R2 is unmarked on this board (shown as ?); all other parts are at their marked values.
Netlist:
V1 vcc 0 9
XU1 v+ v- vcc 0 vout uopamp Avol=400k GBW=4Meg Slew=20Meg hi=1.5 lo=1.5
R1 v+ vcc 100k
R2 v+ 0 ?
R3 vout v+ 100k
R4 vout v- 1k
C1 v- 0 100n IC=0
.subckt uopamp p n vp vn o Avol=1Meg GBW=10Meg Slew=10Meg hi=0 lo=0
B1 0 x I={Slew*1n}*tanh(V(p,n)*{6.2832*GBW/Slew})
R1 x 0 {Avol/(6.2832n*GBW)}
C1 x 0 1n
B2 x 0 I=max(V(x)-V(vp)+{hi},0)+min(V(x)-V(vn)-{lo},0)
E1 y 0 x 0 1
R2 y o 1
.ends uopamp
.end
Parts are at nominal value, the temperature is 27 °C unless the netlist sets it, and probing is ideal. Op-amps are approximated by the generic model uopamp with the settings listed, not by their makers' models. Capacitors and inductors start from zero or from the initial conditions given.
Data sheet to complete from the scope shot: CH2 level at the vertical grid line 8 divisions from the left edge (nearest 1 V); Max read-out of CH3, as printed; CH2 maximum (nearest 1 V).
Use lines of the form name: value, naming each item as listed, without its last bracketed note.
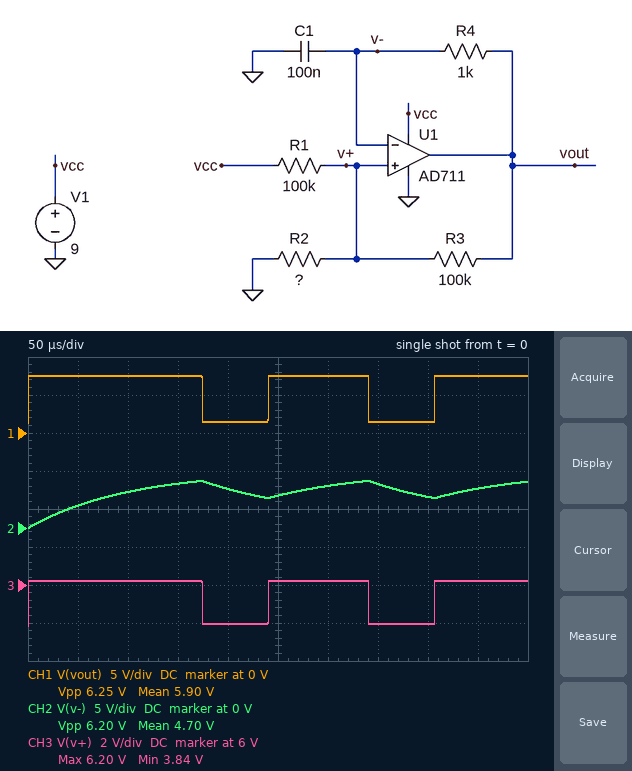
CH2 level at the vertical grid line 8 divisions from the left edge: 4 V
Max read-out of CH3, as printed: 6.20 V
CH2 maximum: 6 V
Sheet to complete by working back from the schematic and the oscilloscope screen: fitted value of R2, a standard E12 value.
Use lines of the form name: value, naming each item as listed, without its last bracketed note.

fitted value of R2, a standard E12 value: 150 kΩ
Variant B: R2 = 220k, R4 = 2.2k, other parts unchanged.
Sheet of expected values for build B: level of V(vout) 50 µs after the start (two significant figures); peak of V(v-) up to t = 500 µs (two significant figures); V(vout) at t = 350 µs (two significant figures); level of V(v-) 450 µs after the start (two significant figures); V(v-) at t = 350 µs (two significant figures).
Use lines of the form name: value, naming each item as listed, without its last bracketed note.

level of V(vout) 50 µs after the start: 7.5 V
peak of V(v-) up to t = 500 µs: 6.7 V
V(vout) at t = 350 µs: 7.5 V
level of V(v-) 450 µs after the start: 6.5 V
V(v-) at t = 350 µs: 6.0 V
